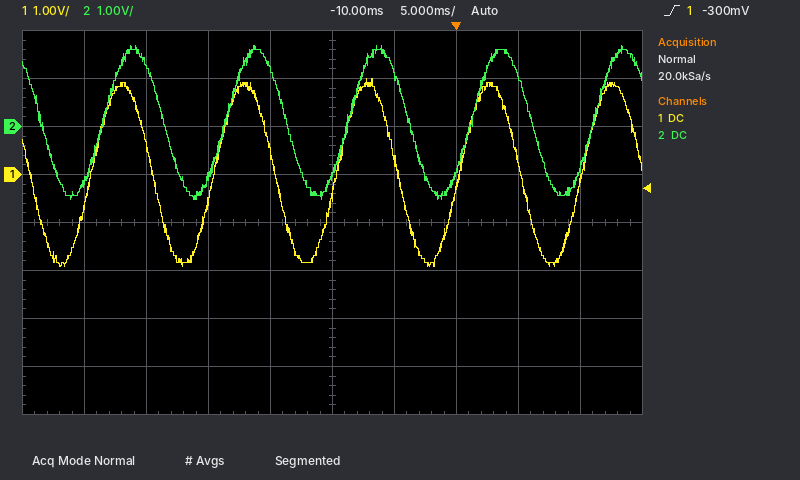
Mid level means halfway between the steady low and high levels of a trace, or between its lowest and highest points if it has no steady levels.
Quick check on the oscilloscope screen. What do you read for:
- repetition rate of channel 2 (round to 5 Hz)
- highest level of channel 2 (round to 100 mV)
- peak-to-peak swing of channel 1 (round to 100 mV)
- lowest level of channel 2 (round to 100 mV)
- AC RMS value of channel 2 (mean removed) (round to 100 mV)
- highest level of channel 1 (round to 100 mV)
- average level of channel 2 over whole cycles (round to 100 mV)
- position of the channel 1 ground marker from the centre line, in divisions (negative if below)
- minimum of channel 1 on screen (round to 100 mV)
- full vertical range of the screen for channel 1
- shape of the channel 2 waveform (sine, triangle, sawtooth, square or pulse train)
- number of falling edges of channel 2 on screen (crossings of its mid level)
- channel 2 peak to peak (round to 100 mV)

100 Hz
1.7 V
3.9 V
-1.5 V
1.1 V
2.0 V
100 mV
+1.0 div
-1.9 V
8 V
sine
5
3.2 V
